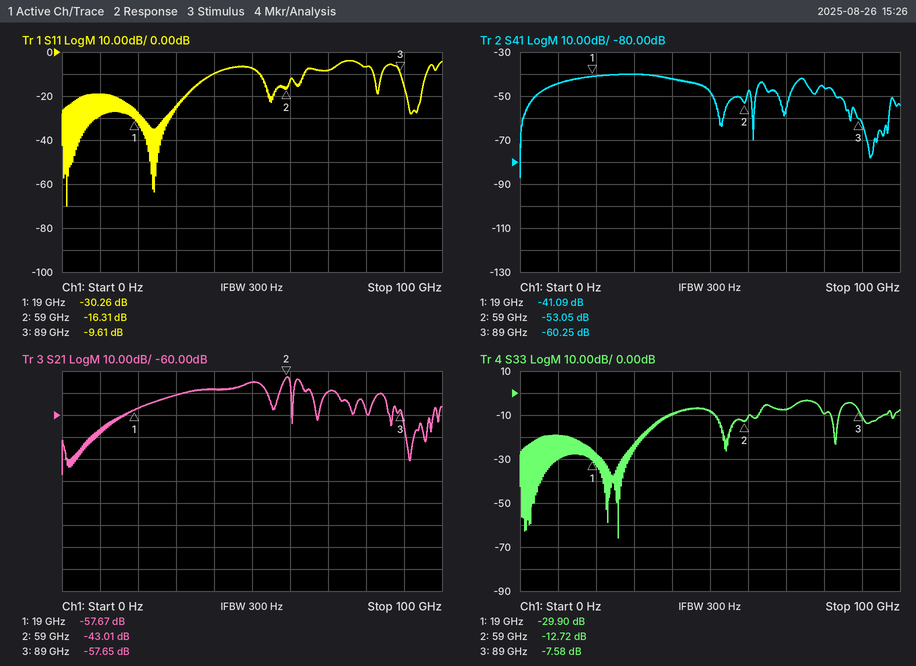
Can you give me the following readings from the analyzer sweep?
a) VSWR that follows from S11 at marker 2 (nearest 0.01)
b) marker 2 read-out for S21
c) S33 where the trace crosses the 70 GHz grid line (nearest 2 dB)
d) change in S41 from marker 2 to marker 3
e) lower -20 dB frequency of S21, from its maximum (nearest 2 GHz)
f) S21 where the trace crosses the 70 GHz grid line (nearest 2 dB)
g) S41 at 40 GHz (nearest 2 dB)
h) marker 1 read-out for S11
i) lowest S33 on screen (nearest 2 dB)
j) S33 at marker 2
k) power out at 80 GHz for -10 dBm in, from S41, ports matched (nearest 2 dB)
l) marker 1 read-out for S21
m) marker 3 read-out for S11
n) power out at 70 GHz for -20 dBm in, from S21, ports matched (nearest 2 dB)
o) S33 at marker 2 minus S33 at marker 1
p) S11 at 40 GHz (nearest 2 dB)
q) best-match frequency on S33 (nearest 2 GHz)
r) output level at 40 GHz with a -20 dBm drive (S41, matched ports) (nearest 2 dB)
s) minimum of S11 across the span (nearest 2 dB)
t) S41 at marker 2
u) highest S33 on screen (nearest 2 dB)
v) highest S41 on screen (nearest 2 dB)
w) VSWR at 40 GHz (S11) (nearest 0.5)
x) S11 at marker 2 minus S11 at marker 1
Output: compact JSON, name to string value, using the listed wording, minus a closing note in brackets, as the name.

{"VSWR that follows from S11 at marker 2": "1.36", "marker 2 read-out for S21": "-43.01 dB", "S33 where the trace crosses the 70 GHz grid line": "-8 dB", "change in S41 from marker 2 to marker 3": "-7.20 dB", "lower -20 dB frequency of S21, from its maximum": "14 GHz", "S21 where the trace crosses the 70 GHz grid line": "-50 dB", "S41 at 40 GHz": "-42 dB", "marker 1 read-out for S11": "-30.26 dB", "lowest S33 on screen": "-66 dB", "S33 at marker 2": "-12.72 dB", "power out at 80 GHz for -10 dBm in, from S41, ports matched": "-56 dBm", "marker 1 read-out for S21": "-57.67 dB", "marker 3 read-out for S11": "-9.61 dB", "power out at 70 GHz for -20 dBm in, from S21, ports matched": "-70 dBm", "S33 at marker 2 minus S33 at marker 1": "17.18 dB", "S11 at 40 GHz": "-10 dB", "best-match frequency on S33": "26 GHz", "output level at 40 GHz with a -20 dBm drive (S41, matched ports)": "-62 dBm", "minimum of S11 across the span": "-70 dB", "S41 at marker 2": "-53.05 dB", "highest S33 on screen": "-4 dB", "highest S41 on screen": "-40 dB", "VSWR at 40 GHz (S11)": "2.0", "S11 at marker 2 minus S11 at marker 1": "13.95 dB"}
